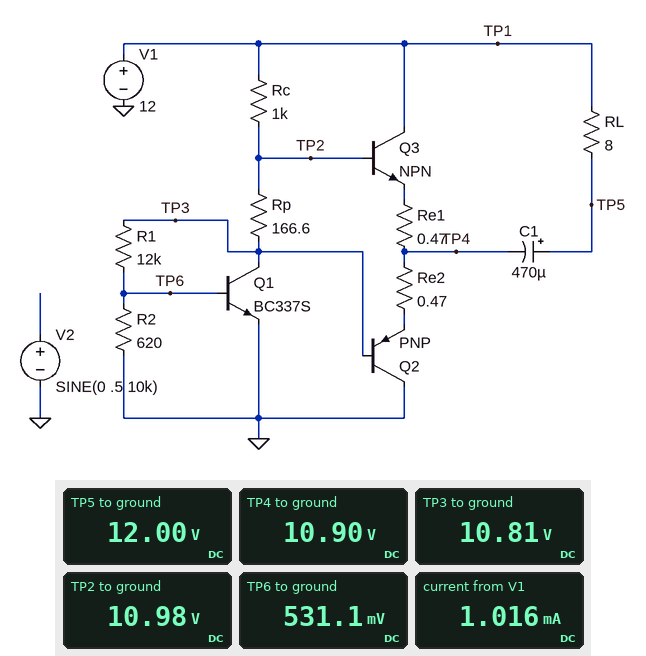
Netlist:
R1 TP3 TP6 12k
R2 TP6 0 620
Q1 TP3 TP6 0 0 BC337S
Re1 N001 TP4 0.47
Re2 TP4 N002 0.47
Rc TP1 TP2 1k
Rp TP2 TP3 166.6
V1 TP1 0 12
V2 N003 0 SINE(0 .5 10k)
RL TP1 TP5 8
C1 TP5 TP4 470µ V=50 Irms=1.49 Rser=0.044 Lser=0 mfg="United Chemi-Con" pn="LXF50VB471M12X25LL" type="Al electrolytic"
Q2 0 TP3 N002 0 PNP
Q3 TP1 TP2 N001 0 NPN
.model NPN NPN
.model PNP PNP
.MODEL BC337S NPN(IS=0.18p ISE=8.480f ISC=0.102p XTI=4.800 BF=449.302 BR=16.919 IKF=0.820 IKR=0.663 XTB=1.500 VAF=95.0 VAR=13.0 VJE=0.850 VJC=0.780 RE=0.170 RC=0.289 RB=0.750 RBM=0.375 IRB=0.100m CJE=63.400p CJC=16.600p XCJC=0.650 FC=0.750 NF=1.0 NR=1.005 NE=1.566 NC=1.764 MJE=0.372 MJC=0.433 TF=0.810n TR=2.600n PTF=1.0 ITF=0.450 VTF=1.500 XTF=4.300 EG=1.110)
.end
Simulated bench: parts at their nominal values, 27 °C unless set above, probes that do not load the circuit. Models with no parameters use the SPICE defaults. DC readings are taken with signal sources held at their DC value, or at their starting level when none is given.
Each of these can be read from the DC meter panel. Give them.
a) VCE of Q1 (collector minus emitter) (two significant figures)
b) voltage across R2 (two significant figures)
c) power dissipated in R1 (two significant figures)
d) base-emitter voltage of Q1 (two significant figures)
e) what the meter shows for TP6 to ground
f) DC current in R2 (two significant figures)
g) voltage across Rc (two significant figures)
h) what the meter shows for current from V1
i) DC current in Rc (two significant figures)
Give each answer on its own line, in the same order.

11 V
530 mV
8.8 mW
530 mV
531.1 mV
860 µA
1.0 V
1.016 mA
1.0 mA
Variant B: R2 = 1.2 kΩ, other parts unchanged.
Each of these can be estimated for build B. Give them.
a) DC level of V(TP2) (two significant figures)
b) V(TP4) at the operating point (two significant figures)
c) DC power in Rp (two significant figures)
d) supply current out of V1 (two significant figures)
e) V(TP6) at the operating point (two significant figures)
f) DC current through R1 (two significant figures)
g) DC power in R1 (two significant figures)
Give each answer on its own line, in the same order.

7.6 V
7.2 V
3.2 mW
4.4 mA
620 mV
520 µA
3.3 mW
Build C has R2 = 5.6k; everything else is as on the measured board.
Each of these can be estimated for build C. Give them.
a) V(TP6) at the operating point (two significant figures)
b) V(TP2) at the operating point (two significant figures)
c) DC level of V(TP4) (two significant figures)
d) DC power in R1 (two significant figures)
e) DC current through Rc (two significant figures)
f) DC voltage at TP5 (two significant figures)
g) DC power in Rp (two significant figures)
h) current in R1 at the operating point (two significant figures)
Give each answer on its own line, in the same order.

640 mV
3.6 V
2.9 V
210 µW
8.4 mA
12 V
12 mW
130 µA
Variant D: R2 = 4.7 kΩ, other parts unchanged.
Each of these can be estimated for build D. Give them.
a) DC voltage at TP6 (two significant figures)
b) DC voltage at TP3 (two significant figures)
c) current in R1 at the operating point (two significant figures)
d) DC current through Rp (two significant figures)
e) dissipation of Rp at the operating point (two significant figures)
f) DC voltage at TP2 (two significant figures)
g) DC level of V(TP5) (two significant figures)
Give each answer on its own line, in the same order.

640 mV
2.5 V
150 µA
8.2 mA
11 mW
3.8 V
12 V
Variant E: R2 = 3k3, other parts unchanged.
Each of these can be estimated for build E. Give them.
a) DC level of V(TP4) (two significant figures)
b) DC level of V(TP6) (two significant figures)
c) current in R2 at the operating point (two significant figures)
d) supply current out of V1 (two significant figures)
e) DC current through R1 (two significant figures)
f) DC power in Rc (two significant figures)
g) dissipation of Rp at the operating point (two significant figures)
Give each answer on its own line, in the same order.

3.8 V
630 mV
190 µA
7.6 mA
210 µA
58 mW
9.6 mW
